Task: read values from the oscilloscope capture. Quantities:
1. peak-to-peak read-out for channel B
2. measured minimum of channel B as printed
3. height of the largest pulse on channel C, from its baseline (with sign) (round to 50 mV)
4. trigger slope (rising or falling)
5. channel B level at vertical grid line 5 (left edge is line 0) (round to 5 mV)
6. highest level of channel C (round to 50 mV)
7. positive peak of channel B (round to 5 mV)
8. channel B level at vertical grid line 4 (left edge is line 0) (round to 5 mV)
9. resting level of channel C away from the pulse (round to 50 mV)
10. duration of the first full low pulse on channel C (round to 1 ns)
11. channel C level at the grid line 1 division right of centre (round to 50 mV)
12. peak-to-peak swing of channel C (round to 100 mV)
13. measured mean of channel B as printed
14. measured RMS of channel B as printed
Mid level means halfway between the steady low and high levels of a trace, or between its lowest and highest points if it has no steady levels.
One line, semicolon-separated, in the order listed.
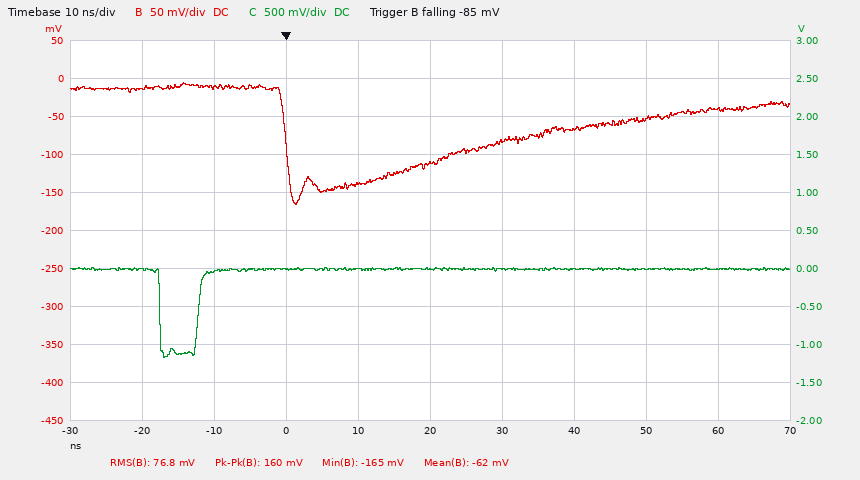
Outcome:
160 mV; -165 mV; -1.15 V; falling; -110 mV; 0 mV; -5 mV; -140 mV; 0 mV; 5 ns; 0 mV; 1.20 V; -62 mV; 76.8 mV
